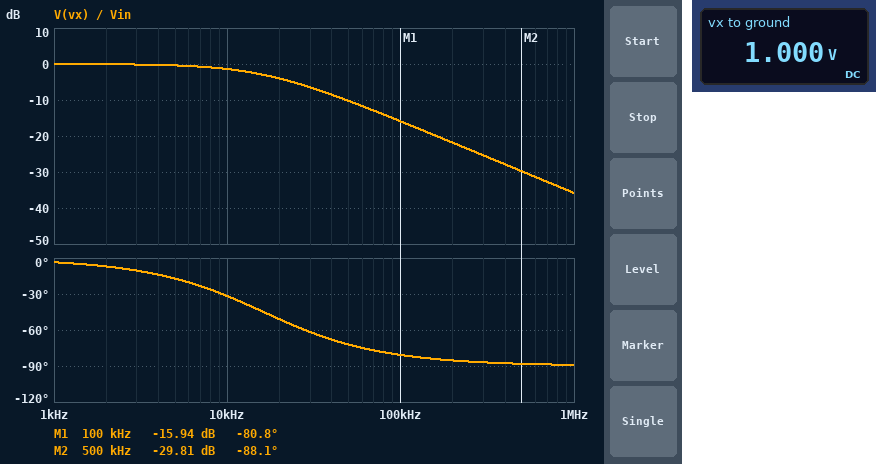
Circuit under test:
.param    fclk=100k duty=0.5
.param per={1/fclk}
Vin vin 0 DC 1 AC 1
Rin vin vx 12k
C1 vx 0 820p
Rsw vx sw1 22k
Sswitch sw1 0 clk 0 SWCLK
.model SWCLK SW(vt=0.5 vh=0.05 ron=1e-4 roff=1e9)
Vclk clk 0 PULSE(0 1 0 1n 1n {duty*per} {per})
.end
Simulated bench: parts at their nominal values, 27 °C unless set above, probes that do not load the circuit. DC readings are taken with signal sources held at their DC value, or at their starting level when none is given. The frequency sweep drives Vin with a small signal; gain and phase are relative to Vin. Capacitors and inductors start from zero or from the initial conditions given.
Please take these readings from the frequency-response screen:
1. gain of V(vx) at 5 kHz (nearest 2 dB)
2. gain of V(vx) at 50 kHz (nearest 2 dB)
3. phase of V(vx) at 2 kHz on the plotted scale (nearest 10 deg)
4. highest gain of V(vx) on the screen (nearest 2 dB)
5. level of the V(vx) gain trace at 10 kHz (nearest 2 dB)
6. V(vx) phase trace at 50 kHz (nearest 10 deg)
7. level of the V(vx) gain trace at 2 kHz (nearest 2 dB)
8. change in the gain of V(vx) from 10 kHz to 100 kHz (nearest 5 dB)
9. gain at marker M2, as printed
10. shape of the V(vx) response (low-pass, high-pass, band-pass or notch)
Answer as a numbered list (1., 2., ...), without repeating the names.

1. 0 dB
2. -10 dB
3. -10 deg
4. 0 dB
5. -2 dB
6. -70 deg
7. 0 dB
8. -15 dB
9. -29.81 dB
10. low-pass
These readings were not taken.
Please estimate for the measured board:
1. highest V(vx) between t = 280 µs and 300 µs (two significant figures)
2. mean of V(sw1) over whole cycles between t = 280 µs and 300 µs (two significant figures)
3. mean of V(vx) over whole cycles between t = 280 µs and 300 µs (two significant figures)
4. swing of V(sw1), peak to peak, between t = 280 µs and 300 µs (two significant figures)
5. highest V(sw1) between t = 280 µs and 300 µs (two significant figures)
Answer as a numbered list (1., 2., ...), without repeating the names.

1. 840 mV
2. 400 mV
3. 790 mV
4. 840 mV
5. 840 mV
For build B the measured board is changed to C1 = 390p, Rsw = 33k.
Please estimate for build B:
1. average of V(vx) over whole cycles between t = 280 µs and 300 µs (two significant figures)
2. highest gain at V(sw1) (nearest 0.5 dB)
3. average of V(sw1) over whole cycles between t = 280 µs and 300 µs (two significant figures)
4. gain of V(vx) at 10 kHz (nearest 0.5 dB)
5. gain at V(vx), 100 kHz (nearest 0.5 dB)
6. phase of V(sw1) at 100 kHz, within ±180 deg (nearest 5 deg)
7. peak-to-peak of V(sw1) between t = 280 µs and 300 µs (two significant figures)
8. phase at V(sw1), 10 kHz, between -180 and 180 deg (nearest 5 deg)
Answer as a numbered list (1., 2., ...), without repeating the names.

1. 850 mV
2. 0 dB
3. 430 mV
4. -0.5 dB
5. -10.0 dB
6. -70 deg
7. 920 mV
8. -15 deg
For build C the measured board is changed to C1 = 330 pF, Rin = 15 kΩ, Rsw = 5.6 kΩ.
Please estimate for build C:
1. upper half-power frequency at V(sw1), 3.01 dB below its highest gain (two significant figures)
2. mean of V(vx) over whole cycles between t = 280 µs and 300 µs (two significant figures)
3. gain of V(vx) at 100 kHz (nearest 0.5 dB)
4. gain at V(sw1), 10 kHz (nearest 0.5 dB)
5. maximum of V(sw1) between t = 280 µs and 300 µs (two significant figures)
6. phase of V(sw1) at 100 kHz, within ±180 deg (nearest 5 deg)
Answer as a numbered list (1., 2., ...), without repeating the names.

1. 32 kHz
2. 470 mV
3. -10.5 dB
4. -0.5 dB
5. 740 mV
6. -70 deg
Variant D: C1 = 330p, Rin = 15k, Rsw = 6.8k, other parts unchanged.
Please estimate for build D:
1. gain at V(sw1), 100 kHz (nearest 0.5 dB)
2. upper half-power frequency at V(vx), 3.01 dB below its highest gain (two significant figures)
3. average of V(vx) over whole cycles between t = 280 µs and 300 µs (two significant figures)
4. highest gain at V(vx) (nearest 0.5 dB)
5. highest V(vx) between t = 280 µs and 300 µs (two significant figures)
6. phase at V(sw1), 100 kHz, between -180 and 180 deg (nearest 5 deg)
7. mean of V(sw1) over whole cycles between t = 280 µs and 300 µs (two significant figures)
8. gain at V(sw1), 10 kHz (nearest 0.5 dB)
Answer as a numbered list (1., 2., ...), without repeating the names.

1. -10.5 dB
2. 32 kHz
3. 510 mV
4. 0 dB
5. 760 mV
6. -70 deg
7. 290 mV
8. -0.5 dB
